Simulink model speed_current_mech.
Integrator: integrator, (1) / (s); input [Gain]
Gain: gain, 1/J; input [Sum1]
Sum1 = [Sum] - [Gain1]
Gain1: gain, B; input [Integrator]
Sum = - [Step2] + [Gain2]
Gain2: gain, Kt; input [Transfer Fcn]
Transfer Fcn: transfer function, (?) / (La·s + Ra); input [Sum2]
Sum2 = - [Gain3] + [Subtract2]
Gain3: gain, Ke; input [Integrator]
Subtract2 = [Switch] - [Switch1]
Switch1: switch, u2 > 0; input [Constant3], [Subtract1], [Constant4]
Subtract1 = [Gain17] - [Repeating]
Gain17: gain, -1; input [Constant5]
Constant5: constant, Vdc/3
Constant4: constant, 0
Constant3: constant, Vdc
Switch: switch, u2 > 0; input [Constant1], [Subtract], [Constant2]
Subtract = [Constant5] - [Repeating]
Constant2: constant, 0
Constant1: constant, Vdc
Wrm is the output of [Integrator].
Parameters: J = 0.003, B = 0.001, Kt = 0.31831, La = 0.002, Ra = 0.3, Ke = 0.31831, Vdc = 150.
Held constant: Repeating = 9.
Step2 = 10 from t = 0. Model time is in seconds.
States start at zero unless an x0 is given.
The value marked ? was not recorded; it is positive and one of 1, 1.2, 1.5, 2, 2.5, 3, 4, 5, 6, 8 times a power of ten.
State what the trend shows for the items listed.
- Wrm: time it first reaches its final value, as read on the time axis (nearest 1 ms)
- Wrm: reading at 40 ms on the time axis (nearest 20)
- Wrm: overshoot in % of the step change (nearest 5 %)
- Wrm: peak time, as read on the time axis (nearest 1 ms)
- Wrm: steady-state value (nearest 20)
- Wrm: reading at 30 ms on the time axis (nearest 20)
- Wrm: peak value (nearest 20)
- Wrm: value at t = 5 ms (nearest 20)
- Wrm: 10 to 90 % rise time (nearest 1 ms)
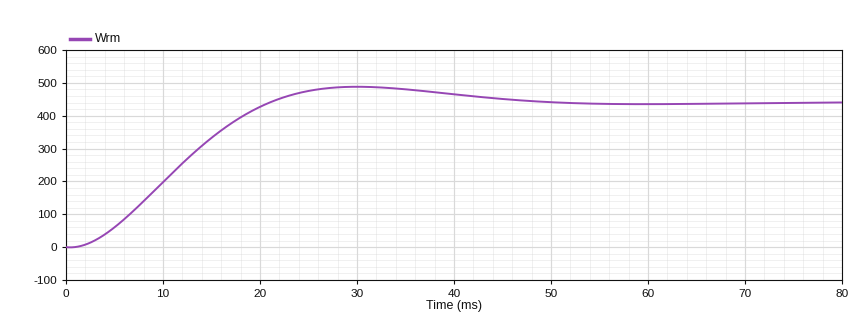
21 ms
460
10 %
30 ms
440
480
480
60
14 ms
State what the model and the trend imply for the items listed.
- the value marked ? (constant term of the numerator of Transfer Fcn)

1
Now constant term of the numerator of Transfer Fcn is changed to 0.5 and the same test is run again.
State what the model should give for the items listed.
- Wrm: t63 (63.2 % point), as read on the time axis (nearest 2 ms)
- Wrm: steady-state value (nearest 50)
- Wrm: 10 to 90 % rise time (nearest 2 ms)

22 ms
400
28 ms
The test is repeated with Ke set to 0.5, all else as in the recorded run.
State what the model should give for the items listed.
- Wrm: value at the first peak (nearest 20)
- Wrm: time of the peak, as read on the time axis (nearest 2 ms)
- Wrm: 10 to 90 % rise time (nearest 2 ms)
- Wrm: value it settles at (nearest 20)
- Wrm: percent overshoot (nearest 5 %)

340
22 ms
10 ms
280
20 %
